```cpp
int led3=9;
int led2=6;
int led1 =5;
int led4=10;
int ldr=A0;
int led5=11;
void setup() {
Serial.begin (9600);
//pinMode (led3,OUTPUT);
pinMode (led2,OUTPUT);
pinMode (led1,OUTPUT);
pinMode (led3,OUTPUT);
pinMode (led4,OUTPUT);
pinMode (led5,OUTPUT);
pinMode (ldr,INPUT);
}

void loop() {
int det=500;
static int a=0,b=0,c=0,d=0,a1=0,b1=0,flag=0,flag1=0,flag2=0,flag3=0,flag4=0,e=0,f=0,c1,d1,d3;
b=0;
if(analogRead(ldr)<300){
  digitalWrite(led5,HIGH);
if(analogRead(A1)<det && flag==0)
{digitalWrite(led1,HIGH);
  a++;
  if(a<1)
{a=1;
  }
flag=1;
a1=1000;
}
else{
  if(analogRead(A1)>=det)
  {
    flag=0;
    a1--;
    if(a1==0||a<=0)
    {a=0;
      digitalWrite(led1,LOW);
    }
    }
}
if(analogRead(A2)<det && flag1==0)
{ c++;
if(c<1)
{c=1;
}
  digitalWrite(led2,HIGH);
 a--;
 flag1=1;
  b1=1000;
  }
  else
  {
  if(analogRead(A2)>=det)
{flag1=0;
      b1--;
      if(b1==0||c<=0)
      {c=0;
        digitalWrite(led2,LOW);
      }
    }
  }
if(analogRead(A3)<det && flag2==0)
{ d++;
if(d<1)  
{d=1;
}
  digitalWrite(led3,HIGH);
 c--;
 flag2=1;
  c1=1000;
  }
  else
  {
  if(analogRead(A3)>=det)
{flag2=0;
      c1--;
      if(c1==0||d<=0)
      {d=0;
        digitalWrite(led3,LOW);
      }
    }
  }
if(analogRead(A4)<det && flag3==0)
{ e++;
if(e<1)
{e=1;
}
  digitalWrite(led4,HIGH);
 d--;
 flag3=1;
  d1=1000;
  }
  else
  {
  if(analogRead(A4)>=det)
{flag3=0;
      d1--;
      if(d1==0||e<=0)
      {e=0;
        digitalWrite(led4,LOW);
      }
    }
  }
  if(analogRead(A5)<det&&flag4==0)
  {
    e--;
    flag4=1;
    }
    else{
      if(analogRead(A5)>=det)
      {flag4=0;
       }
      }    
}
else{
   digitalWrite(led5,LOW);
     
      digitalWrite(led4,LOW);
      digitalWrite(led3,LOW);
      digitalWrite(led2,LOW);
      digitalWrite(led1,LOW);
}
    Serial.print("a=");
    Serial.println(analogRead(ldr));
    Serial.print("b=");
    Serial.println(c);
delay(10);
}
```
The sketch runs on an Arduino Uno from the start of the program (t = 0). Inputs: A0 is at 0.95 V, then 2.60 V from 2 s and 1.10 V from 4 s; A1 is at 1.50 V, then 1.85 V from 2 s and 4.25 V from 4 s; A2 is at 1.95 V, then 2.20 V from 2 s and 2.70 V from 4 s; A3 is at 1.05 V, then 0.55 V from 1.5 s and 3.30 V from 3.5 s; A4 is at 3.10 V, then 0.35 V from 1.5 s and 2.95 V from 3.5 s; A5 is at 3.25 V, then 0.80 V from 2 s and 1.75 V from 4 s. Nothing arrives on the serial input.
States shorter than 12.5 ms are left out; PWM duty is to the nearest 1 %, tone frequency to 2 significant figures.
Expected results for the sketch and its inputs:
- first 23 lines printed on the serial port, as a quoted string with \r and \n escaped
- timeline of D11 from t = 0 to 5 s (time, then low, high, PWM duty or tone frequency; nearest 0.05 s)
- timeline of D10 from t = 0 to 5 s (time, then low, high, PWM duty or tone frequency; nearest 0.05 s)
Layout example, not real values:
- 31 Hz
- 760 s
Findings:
- "a=194\r\nb=0\r\na=194\r\nb=0\r\na=194\r\nb=0\r\na=194\r\nb=0\r\na=194\r\nb=0\r\na=194\r\nb=0\r\na=194\r\nb=0\r\na=194\r\nb=0\r\na=194\r\nb=0\r\na=194\r\nb=0\r\na=194\r\nb=0\r\na=194\r\n"
- 0 s high; 2 s low; 4 s high
- 0 s low; 1.5 s high; 2 s low
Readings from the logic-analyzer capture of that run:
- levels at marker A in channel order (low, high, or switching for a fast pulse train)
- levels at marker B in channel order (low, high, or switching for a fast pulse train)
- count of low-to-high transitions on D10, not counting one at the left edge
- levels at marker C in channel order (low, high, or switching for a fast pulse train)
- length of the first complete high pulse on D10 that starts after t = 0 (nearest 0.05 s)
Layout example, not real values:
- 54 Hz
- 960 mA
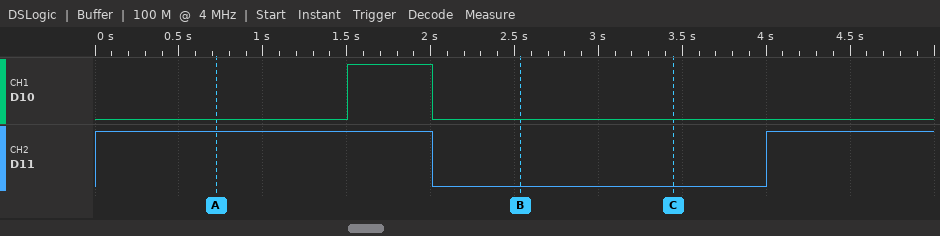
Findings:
- D10 low, D11 high
- D10 low, D11 low
- 1
- D10 low, D11 low
- 0.50 s
